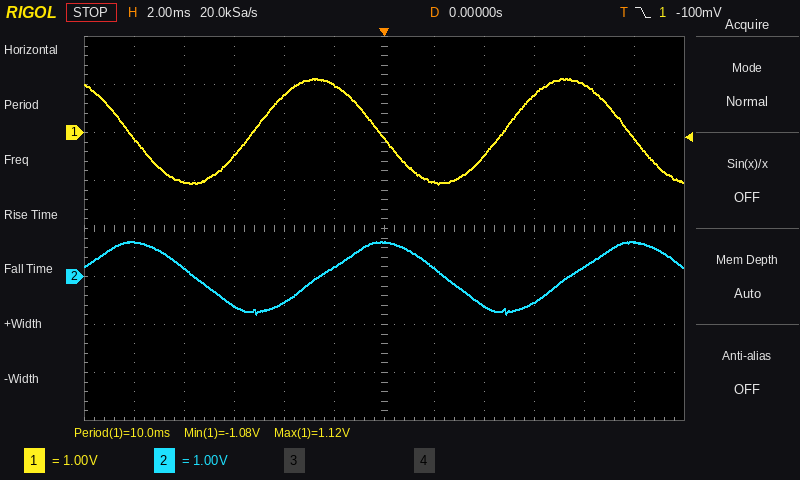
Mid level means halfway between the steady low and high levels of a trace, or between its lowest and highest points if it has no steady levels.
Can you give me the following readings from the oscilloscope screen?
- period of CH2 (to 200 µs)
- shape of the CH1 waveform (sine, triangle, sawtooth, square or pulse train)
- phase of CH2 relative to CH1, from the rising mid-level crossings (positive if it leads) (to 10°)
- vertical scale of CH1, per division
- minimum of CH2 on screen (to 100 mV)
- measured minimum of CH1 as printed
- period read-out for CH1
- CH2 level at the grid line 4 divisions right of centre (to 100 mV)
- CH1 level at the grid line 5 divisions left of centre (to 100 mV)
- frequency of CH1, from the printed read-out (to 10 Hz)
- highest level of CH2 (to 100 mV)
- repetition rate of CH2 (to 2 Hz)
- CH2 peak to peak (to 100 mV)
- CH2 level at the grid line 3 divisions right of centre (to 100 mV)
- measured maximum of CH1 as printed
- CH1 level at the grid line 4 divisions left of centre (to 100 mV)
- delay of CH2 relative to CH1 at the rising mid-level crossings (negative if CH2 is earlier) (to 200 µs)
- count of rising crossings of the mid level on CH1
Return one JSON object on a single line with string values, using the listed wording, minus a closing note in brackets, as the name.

{"period of CH2": "10.0 ms", "shape of the CH1 waveform": "sine", "phase of CH2 relative to CH1, from the rising mid-level crossings (positive if it leads)": "-90°", "vertical scale of CH1, per division": "1 V", "minimum of CH2 on screen": "-800 mV", "measured minimum of CH1 as printed": "-1.08 V", "period read-out for CH1": "10.0 ms", "CH2 level at the grid line 4 divisions right of centre": "200 mV", "CH1 level at the grid line 5 divisions left of centre": "-100 mV", "frequency of CH1, from the printed read-out": "100 Hz", "highest level of CH2": "700 mV", "repetition rate of CH2": "100 Hz", "CH2 peak to peak": "1.5 V", "CH2 level at the grid line 3 divisions right of centre": "-500 mV", "measured maximum of CH1 as printed": "1.12 V", "CH1 level at the grid line 4 divisions left of centre": "-1.0 V", "delay of CH2 relative to CH1 at the rising mid-level crossings (negative if CH2 is earlier)": "+2.6 ms", "count of rising crossings of the mid level on CH1": "2"}
